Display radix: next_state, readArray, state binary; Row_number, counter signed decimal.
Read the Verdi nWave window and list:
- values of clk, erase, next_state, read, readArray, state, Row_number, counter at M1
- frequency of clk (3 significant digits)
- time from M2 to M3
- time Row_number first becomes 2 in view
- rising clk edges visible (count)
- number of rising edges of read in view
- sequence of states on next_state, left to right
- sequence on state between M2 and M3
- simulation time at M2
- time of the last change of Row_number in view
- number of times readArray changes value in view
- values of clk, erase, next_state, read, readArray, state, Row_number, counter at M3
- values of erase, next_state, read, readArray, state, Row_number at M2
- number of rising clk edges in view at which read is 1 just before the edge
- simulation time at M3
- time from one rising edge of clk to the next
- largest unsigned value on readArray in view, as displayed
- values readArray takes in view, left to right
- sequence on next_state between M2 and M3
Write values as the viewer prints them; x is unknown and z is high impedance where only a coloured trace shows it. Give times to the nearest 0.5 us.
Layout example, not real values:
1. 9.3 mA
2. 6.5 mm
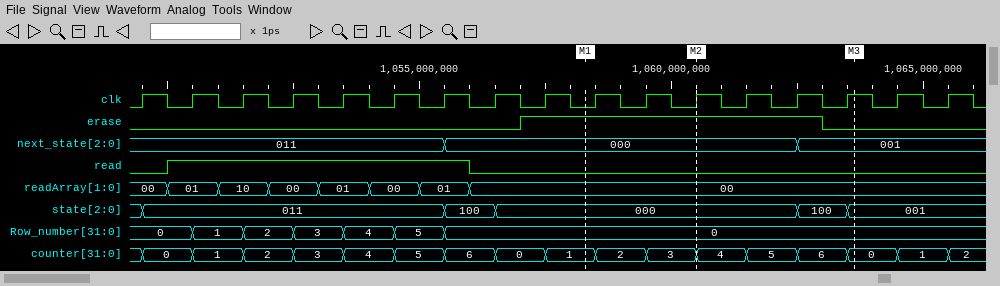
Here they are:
1. clk=0, erase=1, next_state=000, read=0, readArray=00, state=000, Row_number=0, counter=1
2. 1.00 MHz
3. 3 us
4. 1051.5 us
5. 17
6. 1
7. 011, 000, 001
8. 000, 100, 001
9. 1060.5 us
10. 1055.5 us
11. 7
12. clk=1, erase=0, next_state=001, read=0, readArray=00, state=001, Row_number=0, counter=0
13. erase=1, next_state=000, read=0, readArray=00, state=000, Row_number=0
14. 6
15. 1063.5 us
16. 1 us
17. 10
18. 00, 01, 10, 00, 01, 00, 01, 00
19. 000, 001
